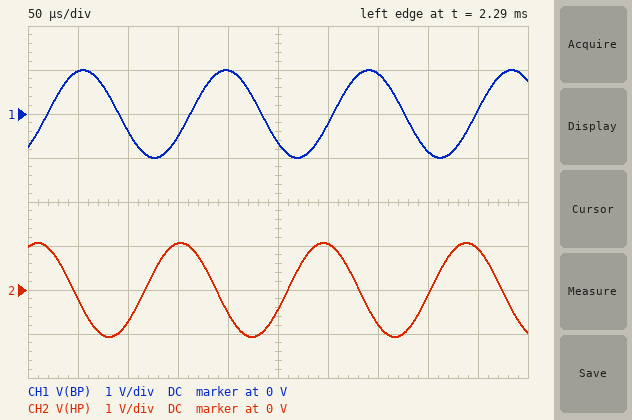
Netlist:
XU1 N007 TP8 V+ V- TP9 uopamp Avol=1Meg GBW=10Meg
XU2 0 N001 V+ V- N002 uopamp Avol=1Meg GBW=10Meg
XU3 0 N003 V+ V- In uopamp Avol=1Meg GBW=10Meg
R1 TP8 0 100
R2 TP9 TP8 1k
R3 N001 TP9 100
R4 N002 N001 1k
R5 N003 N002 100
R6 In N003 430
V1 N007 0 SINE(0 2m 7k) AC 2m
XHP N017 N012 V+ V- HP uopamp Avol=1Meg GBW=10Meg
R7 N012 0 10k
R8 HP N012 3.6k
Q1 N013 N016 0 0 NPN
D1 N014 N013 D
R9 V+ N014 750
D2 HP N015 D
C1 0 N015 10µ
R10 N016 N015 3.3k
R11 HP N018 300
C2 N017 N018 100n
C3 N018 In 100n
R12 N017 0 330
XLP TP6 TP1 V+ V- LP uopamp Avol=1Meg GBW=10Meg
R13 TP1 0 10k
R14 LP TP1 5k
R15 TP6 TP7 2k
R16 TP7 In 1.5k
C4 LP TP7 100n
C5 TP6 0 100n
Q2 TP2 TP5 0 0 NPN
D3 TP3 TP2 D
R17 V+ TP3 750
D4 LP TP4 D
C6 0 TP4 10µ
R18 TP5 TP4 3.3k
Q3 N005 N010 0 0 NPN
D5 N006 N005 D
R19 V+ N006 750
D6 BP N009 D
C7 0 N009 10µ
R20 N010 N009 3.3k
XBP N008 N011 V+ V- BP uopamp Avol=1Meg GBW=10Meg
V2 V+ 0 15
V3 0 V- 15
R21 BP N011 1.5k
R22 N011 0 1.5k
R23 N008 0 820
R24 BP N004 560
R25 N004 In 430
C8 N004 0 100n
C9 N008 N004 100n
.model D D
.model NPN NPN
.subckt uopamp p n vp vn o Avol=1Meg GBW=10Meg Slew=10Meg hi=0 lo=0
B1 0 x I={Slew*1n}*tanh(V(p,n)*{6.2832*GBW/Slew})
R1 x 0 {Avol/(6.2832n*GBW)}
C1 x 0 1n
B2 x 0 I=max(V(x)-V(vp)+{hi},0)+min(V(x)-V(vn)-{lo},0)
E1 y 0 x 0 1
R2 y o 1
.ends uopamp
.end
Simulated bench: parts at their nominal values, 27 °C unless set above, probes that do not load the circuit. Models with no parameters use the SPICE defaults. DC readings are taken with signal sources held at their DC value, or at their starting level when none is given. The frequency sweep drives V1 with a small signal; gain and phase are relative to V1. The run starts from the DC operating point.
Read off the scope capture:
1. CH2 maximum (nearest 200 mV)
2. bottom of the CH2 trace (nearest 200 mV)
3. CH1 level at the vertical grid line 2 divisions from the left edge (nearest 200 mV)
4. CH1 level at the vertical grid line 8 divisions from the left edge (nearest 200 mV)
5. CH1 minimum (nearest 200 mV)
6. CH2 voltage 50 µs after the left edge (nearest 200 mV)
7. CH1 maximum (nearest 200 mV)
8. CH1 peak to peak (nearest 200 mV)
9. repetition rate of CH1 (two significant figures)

1.0 V
-1.0 V
-400 mV
-800 mV
-1.0 V
-200 mV
1.0 V
2.0 V
7.0 kHz
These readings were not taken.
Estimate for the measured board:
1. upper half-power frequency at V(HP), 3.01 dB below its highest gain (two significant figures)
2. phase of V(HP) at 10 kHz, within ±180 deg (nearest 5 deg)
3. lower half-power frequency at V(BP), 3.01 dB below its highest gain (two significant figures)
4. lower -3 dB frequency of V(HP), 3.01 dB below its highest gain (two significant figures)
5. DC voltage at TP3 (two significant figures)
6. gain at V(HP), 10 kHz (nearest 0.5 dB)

540 kHz
45 deg
1.9 kHz
5.5 kHz
15 V
55.5 dB
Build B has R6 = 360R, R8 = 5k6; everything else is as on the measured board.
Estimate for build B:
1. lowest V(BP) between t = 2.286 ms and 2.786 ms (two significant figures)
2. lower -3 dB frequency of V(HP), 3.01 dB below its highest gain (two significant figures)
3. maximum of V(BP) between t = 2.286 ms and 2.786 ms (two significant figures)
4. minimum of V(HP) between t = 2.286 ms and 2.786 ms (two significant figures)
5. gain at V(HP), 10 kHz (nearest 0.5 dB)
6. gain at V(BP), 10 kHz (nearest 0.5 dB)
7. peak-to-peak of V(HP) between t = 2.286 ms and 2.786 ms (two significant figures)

-830 mV
4.8 kHz
830 mV
-1.2 V
56.0 dB
49.5 dB
2.3 V
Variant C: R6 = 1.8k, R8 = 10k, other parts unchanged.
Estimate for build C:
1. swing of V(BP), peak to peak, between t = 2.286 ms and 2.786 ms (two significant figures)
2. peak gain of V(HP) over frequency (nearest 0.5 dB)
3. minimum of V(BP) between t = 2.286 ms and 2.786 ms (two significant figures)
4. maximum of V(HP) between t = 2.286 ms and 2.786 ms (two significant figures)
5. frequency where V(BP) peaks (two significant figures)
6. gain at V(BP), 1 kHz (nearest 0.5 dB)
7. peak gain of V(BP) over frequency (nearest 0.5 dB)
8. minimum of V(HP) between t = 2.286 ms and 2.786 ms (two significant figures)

8.3 V
74.0 dB
-4.2 V
10 V
3.6 kHz
61.5 dB
70.0 dB
-10 V
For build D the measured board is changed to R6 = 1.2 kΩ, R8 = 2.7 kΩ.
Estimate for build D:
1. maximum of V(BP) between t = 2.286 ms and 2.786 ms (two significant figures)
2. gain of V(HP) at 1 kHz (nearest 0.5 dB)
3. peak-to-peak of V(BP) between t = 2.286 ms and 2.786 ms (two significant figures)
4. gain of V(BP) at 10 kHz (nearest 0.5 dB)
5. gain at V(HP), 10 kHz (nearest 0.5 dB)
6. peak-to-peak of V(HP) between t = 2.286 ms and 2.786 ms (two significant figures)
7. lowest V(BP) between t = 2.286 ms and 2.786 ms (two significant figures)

2.8 V
36.0 dB
5.6 V
60.0 dB
63.5 dB
5.3 V
-2.8 V
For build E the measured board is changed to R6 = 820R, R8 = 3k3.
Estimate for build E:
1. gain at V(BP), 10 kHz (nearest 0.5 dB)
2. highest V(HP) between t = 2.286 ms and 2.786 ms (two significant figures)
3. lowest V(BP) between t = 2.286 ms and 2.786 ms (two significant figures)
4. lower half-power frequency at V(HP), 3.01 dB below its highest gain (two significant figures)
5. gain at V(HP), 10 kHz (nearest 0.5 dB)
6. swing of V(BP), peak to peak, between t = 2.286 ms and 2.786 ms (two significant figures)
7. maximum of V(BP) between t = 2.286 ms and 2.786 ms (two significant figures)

56.5 dB
2.0 V
-1.9 V
5.6 kHz
61.0 dB
3.8 V
1.9 V
